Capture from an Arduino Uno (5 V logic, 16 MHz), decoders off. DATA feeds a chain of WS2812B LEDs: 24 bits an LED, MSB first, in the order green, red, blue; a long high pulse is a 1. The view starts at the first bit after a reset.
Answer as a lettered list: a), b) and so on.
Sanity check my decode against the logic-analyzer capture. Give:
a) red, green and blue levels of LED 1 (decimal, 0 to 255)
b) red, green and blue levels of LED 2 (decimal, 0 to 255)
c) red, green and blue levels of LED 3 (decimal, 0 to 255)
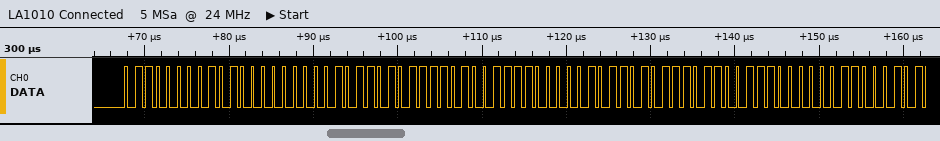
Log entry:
a) 160, 96, 11
b) 158, 94, 11
c) 156, 93, 12
